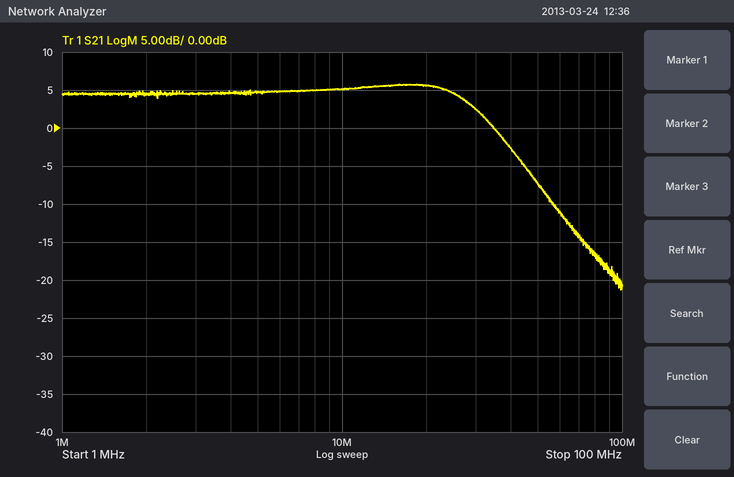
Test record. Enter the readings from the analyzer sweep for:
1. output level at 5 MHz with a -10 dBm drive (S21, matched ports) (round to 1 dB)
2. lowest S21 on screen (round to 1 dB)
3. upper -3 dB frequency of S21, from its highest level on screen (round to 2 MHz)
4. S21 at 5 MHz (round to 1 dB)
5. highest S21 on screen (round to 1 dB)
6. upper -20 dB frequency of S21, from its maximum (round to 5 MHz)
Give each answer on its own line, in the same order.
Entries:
-5 dBm
-21 dB
30 MHz
5 dB
6 dB
70 MHz
